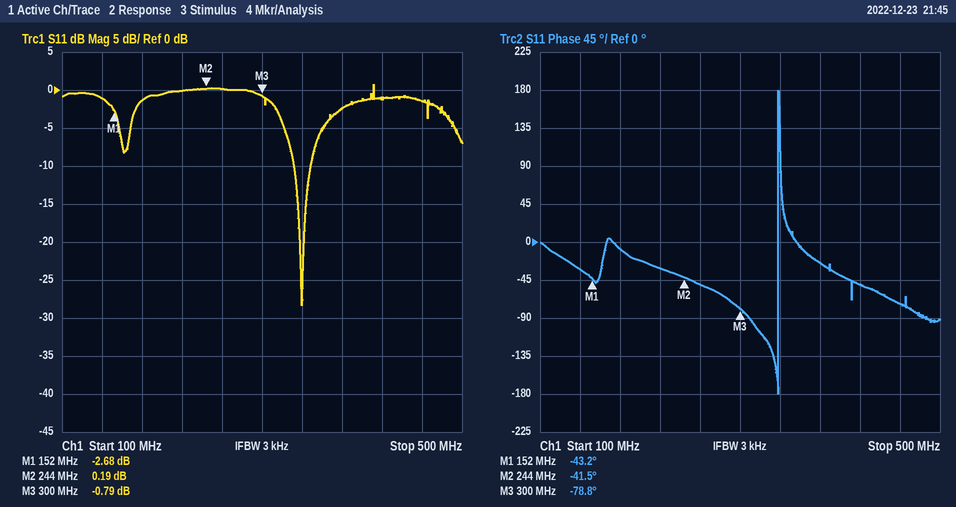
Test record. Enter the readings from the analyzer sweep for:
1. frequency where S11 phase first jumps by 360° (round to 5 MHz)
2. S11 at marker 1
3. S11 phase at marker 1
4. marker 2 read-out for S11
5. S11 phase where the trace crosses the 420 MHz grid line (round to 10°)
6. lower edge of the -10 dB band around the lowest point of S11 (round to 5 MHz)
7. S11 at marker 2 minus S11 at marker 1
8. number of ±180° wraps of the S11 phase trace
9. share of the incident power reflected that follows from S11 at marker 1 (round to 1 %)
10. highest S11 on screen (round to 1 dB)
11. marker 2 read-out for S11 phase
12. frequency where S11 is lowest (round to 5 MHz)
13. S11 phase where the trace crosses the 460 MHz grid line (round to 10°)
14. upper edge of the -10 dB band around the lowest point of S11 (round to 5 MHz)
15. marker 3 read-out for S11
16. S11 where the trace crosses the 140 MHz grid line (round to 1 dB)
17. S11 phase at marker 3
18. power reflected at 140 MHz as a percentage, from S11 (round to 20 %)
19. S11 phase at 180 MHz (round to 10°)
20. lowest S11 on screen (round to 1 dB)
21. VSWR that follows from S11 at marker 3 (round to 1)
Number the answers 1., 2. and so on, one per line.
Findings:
1. 340 MHz
2. -2.68 dB
3. -43.2°
4. 0.19 dB
5. -50°
6. 330 MHz
7. 2.87 dB
8. 1
9. 54 %
10. 1 dB
11. -41.5°
12. 340 MHz
13. -70°
14. 350 MHz
15. -0.79 dB
16. -1 dB
17. -78.8°
18. 80 %
19. -10°
20. -28 dB
21. 22
